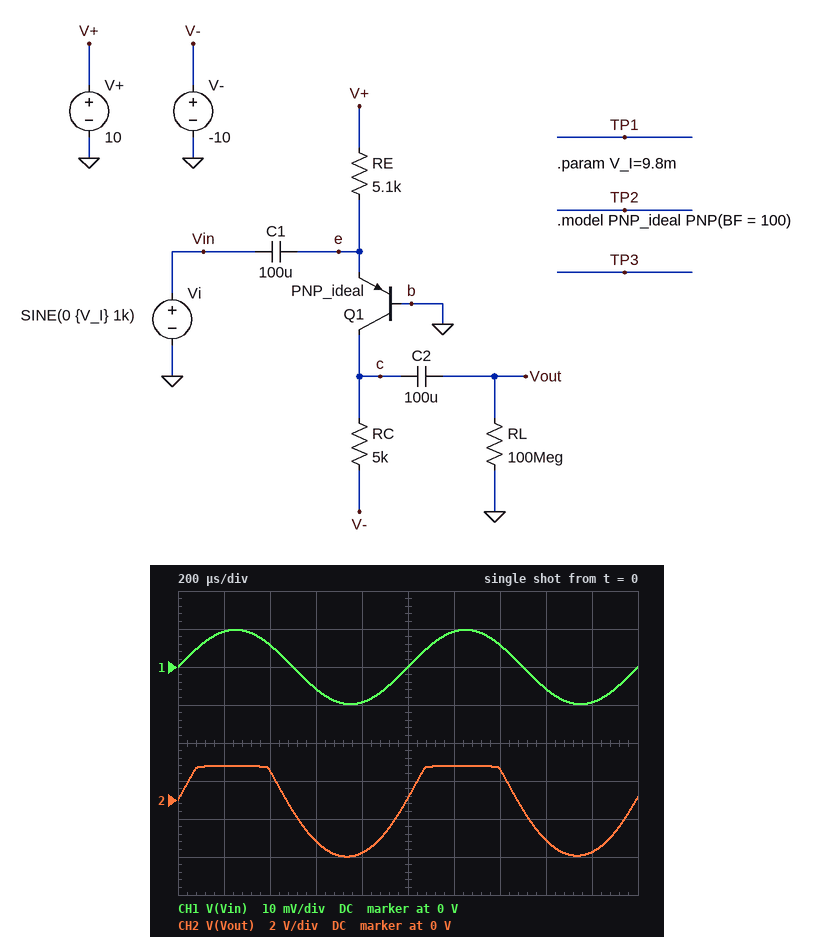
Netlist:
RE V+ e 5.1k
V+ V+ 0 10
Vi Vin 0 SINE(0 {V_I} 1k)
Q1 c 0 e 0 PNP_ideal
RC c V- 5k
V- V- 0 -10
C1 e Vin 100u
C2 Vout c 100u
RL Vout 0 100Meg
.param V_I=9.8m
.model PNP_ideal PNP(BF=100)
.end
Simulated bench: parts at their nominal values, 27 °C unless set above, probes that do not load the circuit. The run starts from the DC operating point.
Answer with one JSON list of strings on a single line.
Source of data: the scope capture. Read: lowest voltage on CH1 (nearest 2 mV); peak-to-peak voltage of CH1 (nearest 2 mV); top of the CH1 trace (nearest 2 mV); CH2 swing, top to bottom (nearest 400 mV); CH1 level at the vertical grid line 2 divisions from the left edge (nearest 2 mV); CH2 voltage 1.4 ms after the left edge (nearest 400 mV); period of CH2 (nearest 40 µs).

["-10 mV", "20 mV", "10 mV", "4.8 V", "6 mV", "1.6 V", "1.00 ms"]
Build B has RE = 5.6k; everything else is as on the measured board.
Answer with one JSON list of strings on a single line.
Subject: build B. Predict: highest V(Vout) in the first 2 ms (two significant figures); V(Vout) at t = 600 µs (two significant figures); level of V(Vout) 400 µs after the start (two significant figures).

["2.6 V", "-2.0 V", "1.4 V"]
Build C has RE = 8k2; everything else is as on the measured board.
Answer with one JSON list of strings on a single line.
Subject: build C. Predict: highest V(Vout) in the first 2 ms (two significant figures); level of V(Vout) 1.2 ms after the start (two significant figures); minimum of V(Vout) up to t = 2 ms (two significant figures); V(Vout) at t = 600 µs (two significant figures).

["2.3 V", "2.2 V", "-1.9 V", "-1.3 V"]
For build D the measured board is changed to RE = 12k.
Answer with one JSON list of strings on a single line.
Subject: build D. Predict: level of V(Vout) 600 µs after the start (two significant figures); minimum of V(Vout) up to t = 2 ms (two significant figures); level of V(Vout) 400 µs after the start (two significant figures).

["-860 mV", "-1.3 V", "780 mV"]
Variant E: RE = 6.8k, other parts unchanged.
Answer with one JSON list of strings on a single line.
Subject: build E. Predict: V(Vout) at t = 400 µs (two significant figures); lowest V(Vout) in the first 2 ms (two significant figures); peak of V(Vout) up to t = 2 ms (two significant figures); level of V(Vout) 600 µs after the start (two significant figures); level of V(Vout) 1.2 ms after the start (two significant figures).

["1.2 V", "-2.3 V", "2.8 V", "-1.6 V", "2.7 V"]
